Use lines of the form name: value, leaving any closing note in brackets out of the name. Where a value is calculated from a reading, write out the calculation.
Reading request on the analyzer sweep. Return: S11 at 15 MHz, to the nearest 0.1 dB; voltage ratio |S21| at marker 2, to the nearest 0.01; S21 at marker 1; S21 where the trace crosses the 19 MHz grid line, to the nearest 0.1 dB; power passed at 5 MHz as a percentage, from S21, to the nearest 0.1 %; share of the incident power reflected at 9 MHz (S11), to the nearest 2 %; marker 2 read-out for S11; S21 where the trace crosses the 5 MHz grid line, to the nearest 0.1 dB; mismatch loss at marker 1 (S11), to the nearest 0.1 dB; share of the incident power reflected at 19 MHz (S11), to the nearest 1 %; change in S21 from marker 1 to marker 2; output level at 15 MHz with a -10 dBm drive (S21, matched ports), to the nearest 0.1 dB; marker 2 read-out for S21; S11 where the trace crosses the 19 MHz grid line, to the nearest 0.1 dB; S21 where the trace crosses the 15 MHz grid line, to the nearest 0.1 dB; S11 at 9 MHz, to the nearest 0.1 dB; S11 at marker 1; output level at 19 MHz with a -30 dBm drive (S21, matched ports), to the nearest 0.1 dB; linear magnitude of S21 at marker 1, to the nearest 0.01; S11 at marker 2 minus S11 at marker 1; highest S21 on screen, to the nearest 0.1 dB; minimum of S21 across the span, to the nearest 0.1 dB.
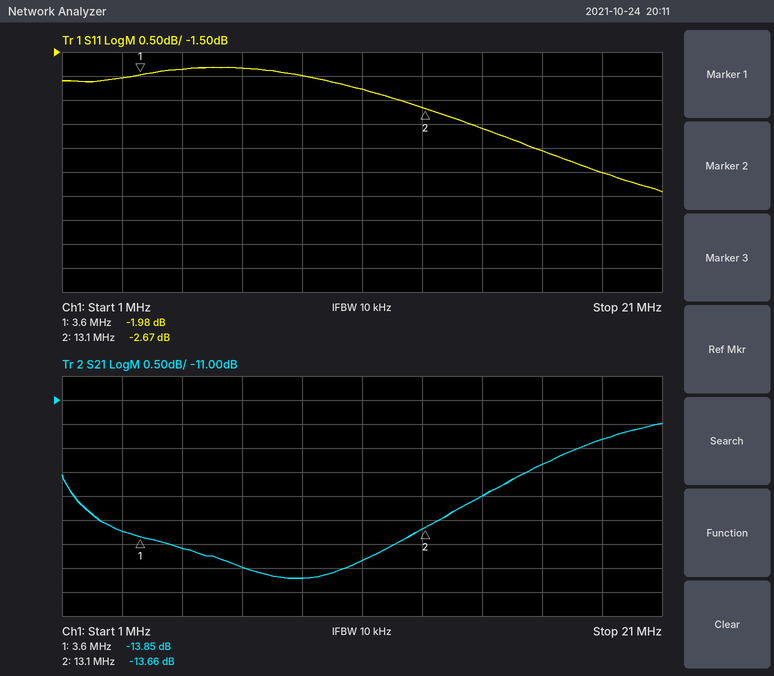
S11 at 15 MHz, to the nearest 0.1 dB: -3.1 dB
voltage ratio |S21| at marker 2, to the nearest 0.01: 10^(-13.66/20) ≈ 0.21
S21 at marker 1: -13.85 dB
S21 where the trace crosses the 19 MHz grid line, to the nearest 0.1 dB: -11.8 dB
power passed at 5 MHz as a percentage, from S21, to the nearest 0.1 %: 10^(-14.1/10) ≈ 3.9 %
share of the incident power reflected at 9 MHz (S11), to the nearest 2 %: 10^(-2/10) ≈ 63.1 %, so 64 % to the nearest 2 %
marker 2 read-out for S11: -2.67 dB
S21 where the trace crosses the 5 MHz grid line, to the nearest 0.1 dB: -14.1 dB
mismatch loss at marker 1 (S11), to the nearest 0.1 dB: −10 log10(1 − 10^(-1.98/10)) ≈ 4.4 dB
share of the incident power reflected at 19 MHz (S11), to the nearest 1 %: 10^(-4/10) ≈ 40 %
change in S21 from marker 1 to marker 2: -13.66 − (-13.85) = 0.19 dB
output level at 15 MHz with a -10 dBm drive (S21, matched ports), to the nearest 0.1 dB: -10 dBm + (-13.0 dB) = -23.0 dBm
marker 2 read-out for S21: -13.66 dB
S11 where the trace crosses the 19 MHz grid line, to the nearest 0.1 dB: -4.0 dB
S21 where the trace crosses the 15 MHz grid line, to the nearest 0.1 dB: -13.0 dB
S11 at 9 MHz, to the nearest 0.1 dB: -2.0 dB
S11 at marker 1: -1.98 dB
output level at 19 MHz with a -30 dBm drive (S21, matched ports), to the nearest 0.1 dB: -30 dBm + (-11.8 dB) = -41.8 dBm
linear magnitude of S21 at marker 1, to the nearest 0.01: 10^(-13.85/20) ≈ 0.20
S11 at marker 2 minus S11 at marker 1: -2.67 − (-1.98) = -0.69 dB
highest S21 on screen, to the nearest 0.1 dB: -11.5 dB
minimum of S21 across the span, to the nearest 0.1 dB: -14.7 dB
